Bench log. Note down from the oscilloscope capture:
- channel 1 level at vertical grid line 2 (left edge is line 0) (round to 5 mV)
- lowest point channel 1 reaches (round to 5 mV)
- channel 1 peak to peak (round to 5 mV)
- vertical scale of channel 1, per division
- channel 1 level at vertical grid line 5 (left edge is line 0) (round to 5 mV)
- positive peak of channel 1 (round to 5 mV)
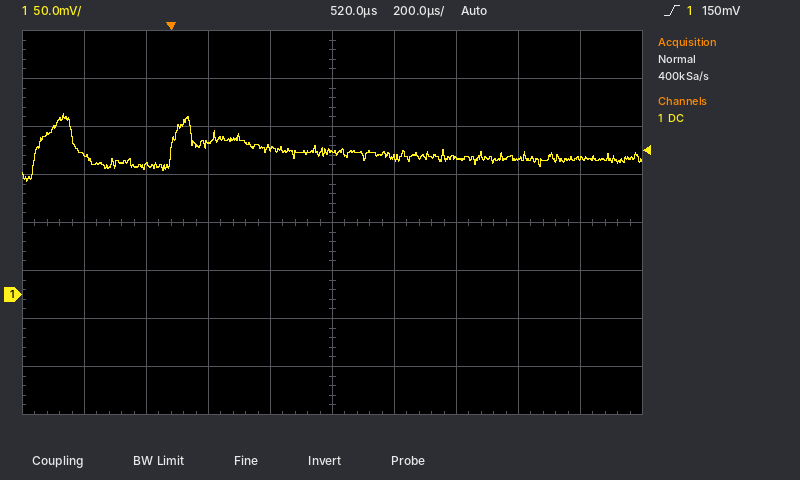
135 mV
120 mV
70 mV
50 mV
150 mV
190 mV
